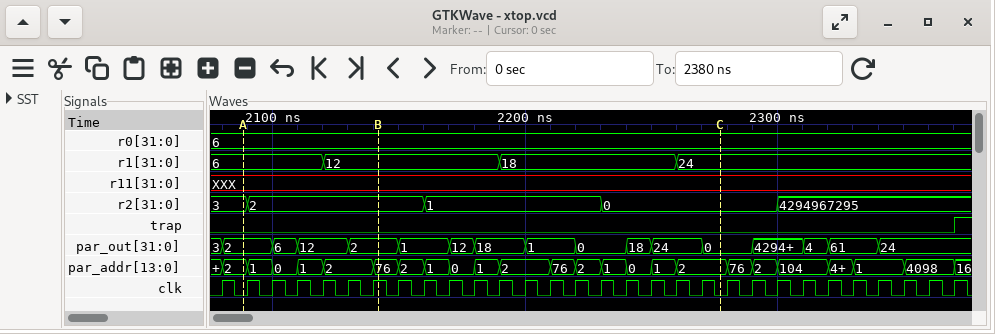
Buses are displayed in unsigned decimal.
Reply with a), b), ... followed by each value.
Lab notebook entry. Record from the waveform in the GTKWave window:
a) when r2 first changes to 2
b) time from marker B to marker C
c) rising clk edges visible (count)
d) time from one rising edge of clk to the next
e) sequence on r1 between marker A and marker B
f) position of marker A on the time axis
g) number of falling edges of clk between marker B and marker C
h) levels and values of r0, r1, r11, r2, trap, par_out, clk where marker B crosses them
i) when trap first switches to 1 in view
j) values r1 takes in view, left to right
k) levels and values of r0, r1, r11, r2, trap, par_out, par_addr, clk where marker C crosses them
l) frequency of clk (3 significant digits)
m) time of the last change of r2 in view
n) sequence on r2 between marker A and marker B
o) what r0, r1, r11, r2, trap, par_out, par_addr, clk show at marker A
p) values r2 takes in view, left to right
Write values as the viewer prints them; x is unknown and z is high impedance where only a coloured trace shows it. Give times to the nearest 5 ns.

a) 2090 ns
b) 135 ns
c) 30
d) 10 ns
e) 6, 12
f) 2090 ns
g) 14
h) r0=6, r1=12, r11=XXX, r2=2, trap=0, par_out=2, clk=1
i) 2370 ns
j) 6, 12, 18, 24
k) r0=6, r1=24, r11=XXX, r2=0, trap=0, par_out=0, par_addr=2, clk=0
l) 100 MHz
m) 2300 ns
n) 3, 2
o) r0=6, r1=6, r11=XXX, r2=3, trap=0, par_out=2, par_addr=2, clk=0
p) 3, 2, 1, 0, 4294967295
